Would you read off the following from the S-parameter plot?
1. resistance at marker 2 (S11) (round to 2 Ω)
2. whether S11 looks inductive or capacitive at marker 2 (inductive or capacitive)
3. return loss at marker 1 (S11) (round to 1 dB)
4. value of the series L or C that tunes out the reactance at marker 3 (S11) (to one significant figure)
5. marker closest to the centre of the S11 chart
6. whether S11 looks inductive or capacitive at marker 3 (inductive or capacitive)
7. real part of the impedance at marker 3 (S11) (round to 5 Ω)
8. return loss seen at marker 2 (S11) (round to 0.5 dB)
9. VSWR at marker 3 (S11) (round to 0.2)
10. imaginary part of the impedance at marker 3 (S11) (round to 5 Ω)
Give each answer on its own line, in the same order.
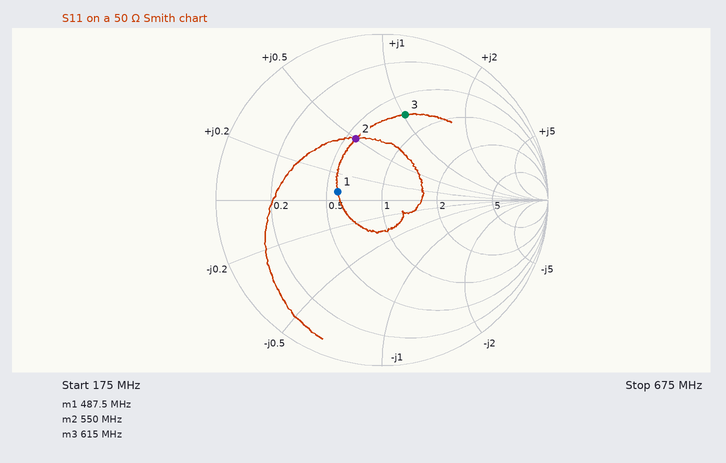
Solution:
28 Ω
inductive
11 dB
5 pF
marker 1
inductive
35 Ω
8.0 dB
3.2
+50 Ω
